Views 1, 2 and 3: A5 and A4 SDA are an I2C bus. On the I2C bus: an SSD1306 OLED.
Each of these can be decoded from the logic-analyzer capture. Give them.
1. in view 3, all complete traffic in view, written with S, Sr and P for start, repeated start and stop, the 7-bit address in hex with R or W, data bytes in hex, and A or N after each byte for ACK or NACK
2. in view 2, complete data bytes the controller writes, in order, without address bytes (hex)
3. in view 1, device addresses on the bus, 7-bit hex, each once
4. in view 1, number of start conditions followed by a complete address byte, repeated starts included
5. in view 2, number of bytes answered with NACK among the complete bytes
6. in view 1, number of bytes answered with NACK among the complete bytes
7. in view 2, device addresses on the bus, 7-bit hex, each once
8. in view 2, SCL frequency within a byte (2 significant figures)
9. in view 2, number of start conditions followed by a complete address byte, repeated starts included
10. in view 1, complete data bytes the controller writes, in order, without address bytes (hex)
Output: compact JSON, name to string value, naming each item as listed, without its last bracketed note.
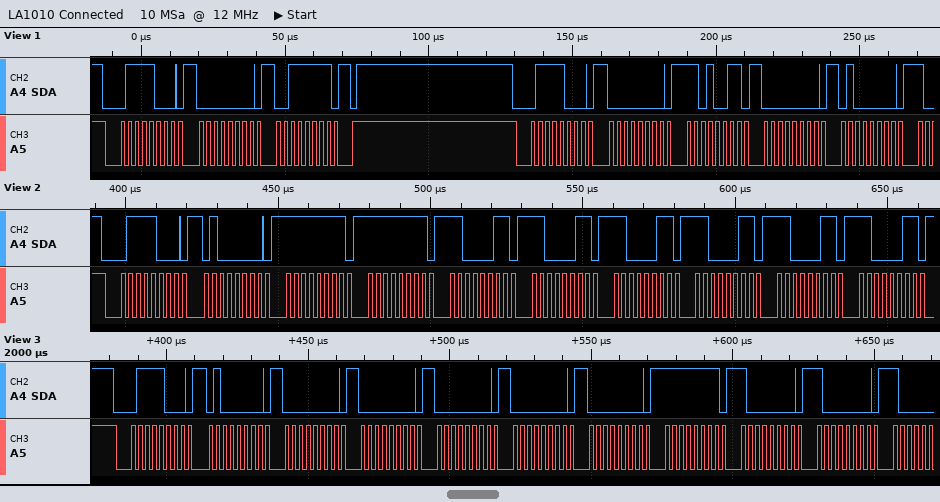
{"in view 3, all complete traffic in view, written with S, Sr and P for start, repeated start and stop, the 7-bit address in hex with R or W, data bytes in hex, and A or N after each byte for ACK or NACK": "S 3CW A 40 A 00 A 00 A 00 A 00 A 00 A FF A 80 A 80 A", "in view 2, complete data bytes the controller writes, in order, without address bytes": "40 FF FF C3 C3 C3 C3 C3 C3", "in view 1, device addresses on the bus, 7-bit hex, each once": "0x3C", "in view 1, number of start conditions followed by a complete address byte, repeated starts included": "2", "in view 2, number of bytes answered with NACK among the complete bytes": "0", "in view 1, number of bytes answered with NACK among the complete bytes": "0", "in view 2, device addresses on the bus, 7-bit hex, each once": "0x3C", "in view 2, SCL frequency within a byte": "400 kHz", "in view 2, number of start conditions followed by a complete address byte, repeated starts included": "1", "in view 1, complete data bytes the controller writes, in order, without address bytes": "00 3F 00 D3 00 40"}
